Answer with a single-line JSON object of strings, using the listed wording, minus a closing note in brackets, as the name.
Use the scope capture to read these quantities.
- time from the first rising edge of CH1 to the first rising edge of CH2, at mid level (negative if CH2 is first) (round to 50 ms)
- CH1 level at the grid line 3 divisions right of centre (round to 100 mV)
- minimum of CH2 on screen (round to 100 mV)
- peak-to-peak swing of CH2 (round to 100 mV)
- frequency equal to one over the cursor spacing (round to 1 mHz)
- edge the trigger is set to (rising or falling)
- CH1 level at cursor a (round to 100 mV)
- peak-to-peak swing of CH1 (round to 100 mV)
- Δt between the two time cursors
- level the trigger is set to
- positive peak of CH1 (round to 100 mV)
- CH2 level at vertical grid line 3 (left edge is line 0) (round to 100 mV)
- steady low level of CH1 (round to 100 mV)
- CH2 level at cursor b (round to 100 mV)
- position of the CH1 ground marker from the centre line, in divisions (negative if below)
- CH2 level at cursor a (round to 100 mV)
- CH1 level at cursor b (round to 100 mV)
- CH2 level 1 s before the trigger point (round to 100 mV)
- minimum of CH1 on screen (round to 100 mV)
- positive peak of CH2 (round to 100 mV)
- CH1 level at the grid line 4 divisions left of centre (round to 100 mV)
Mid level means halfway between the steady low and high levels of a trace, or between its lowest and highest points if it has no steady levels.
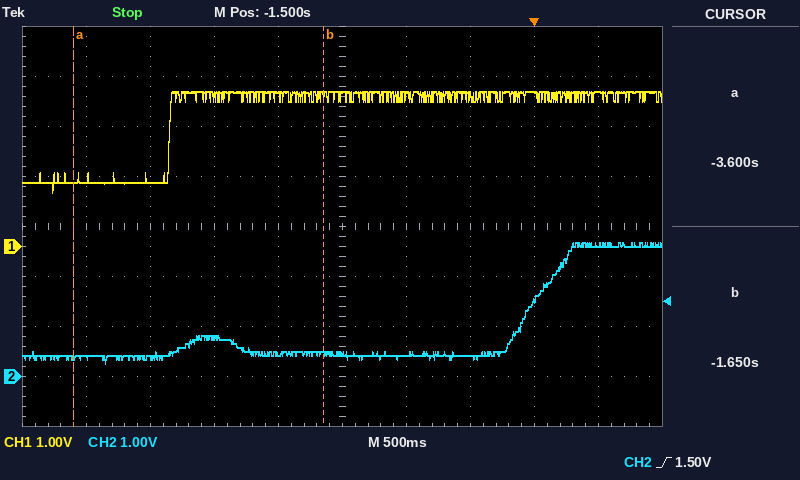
{"time from the first rising edge of CH1 to the first rising edge of CH2, at mid level (negative if CH2 is first)": "+2.85 s", "CH1 level at the grid line 3 divisions right of centre": "3.0 V", "minimum of CH2 on screen": "300 mV", "peak-to-peak swing of CH2": "2.4 V", "frequency equal to one over the cursor spacing": "513 mHz", "edge the trigger is set to": "rising", "CH1 level at cursor a": "1.3 V", "peak-to-peak swing of CH1": "2.0 V", "Δt between the two time cursors": "1.95 s", "level the trigger is set to": "1.50 V", "positive peak of CH1": "3.1 V", "CH2 level at vertical grid line 3 (left edge is line 0)": "800 mV", "steady low level of CH1": "1.3 V", "CH2 level at cursor b": "500 mV", "position of the CH1 ground marker from the centre line, in divisions": "-0.4 div", "CH2 level at cursor a": "400 mV", "CH1 level at cursor b": "3.0 V", "CH2 level 1 s before the trigger point": "400 mV", "minimum of CH1 on screen": "1.1 V", "positive peak of CH2": "2.7 V", "CH1 level at the grid line 4 divisions left of centre": "1.4 V"}
